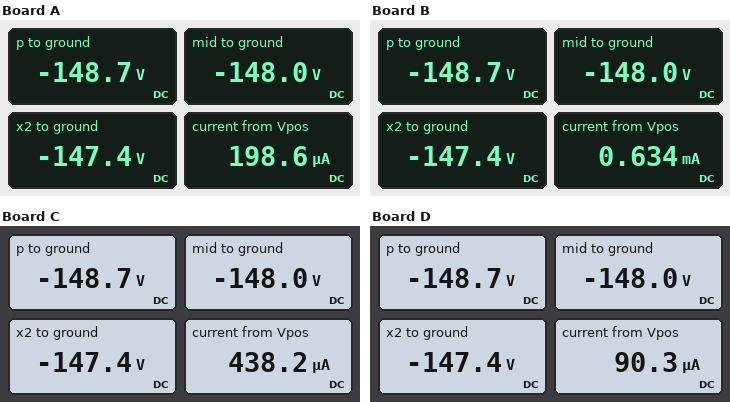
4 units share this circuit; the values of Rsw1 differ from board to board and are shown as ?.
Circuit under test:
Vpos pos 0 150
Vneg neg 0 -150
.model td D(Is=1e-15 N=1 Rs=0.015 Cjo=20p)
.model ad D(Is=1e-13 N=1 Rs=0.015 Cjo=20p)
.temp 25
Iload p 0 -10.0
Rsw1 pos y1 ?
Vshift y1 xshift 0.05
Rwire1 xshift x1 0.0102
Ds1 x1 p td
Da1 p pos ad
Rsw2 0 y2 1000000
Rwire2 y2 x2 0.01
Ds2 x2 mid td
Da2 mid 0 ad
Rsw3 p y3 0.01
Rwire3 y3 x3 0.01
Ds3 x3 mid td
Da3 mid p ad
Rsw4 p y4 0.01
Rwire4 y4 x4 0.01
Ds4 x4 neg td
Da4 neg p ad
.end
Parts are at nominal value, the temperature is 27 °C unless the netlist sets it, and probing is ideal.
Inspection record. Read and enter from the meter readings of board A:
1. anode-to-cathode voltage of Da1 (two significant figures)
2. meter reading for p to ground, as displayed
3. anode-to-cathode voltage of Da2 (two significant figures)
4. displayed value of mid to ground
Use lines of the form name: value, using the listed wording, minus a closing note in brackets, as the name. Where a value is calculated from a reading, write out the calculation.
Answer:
anode-to-cathode voltage of Da1: -148.7 V - 150 V = -300 V
meter reading for p to ground, as displayed: -148.7 V
anode-to-cathode voltage of Da2: -148 V = -150 V
displayed value of mid to ground: -148.0 V
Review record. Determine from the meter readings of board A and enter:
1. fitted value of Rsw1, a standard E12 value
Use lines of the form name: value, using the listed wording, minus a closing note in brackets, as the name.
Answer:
fitted value of Rsw1, a standard E12 value: 1.5 MΩ
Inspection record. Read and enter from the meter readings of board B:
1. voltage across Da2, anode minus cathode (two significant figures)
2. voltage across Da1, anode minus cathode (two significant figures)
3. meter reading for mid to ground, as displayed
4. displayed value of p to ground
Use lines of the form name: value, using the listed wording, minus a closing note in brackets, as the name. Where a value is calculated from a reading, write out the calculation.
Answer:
voltage across Da2, anode minus cathode: -148 V = -150 V
voltage across Da1, anode minus cathode: -148.7 V - 150 V = -300 V
meter reading for mid to ground, as displayed: -148.0 V
displayed value of p to ground: -148.7 V
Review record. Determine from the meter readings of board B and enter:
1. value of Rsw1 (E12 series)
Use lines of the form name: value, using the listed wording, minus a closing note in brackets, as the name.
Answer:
value of Rsw1: 470 kΩ
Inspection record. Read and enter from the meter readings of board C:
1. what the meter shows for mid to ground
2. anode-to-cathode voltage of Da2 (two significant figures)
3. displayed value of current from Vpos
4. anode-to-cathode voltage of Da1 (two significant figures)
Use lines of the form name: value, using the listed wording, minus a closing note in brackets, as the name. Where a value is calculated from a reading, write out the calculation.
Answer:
what the meter shows for mid to ground: -148.0 V
anode-to-cathode voltage of Da2: -148 V = -150 V
displayed value of current from Vpos: 438.2 µA
anode-to-cathode voltage of Da1: -148.7 V - 150 V = -300 V
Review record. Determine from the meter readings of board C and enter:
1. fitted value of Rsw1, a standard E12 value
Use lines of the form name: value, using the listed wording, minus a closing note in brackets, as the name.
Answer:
fitted value of Rsw1, a standard E12 value: 680 kΩ
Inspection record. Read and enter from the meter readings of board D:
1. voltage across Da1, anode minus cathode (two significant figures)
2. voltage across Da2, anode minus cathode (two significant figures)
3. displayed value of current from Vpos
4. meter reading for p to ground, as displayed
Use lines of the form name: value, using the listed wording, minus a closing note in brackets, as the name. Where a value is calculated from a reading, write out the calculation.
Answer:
voltage across Da1, anode minus cathode: -148.7 V - 150 V = -300 V
voltage across Da2, anode minus cathode: -148 V = -150 V
displayed value of current from Vpos: 90.3 µA
meter reading for p to ground, as displayed: -148.7 V
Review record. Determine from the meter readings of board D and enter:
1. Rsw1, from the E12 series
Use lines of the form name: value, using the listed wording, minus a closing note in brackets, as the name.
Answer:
Rsw1, from the E12 series: 3.3 MΩ
